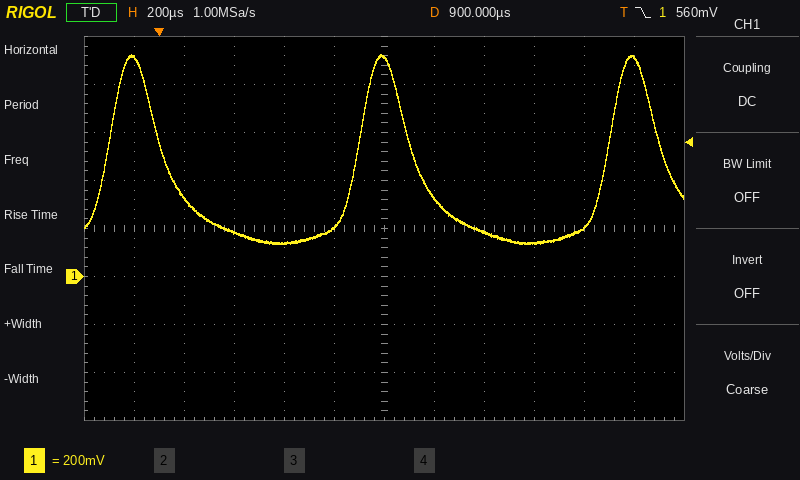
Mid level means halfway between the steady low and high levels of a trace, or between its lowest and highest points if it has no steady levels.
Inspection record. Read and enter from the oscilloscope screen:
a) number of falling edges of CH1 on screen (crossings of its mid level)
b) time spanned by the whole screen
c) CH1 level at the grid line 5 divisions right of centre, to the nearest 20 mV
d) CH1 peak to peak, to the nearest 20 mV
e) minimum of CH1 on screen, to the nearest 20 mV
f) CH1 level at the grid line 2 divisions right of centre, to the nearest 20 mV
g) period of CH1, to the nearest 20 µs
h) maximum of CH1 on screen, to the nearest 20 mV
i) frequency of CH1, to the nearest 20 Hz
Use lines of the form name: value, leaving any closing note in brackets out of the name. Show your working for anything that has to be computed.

number of falling edges of CH1 on screen: 3
time spanned by the whole screen: 2.4 ms
CH1 level at the grid line 5 divisions right of centre, to the nearest 20 mV: 900 mV
CH1 peak to peak, to the nearest 20 mV: 920 mV − (140 mV) = 780 mV
minimum of CH1 on screen, to the nearest 20 mV: 140 mV
CH1 level at the grid line 2 divisions right of centre, to the nearest 20 mV: 180 mV
period of CH1, to the nearest 20 µs: 1.00 ms
maximum of CH1 on screen, to the nearest 20 mV: 920 mV
frequency of CH1, to the nearest 20 Hz: 1 / 1.00 ms ≈ 1.00 kHz
